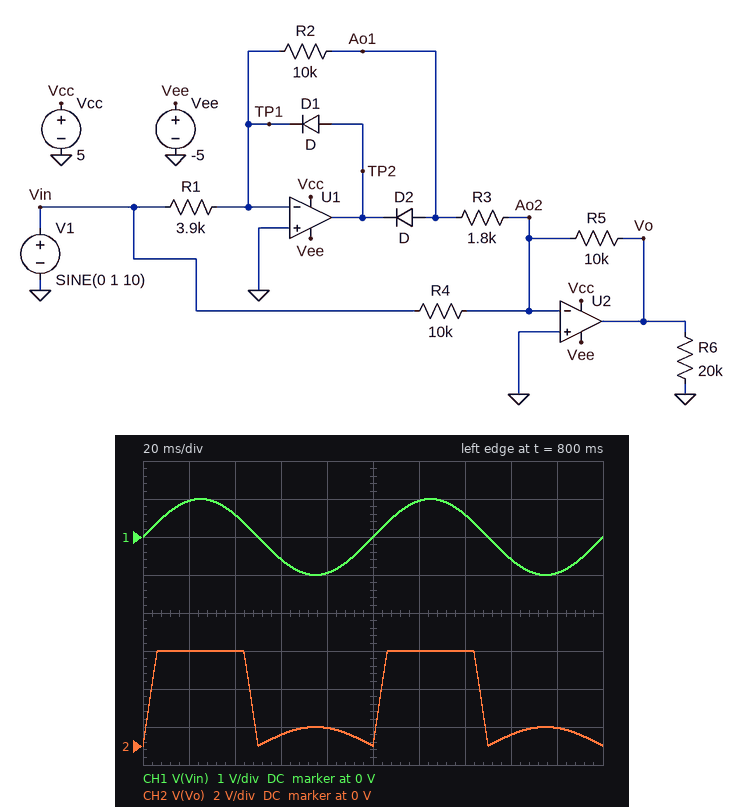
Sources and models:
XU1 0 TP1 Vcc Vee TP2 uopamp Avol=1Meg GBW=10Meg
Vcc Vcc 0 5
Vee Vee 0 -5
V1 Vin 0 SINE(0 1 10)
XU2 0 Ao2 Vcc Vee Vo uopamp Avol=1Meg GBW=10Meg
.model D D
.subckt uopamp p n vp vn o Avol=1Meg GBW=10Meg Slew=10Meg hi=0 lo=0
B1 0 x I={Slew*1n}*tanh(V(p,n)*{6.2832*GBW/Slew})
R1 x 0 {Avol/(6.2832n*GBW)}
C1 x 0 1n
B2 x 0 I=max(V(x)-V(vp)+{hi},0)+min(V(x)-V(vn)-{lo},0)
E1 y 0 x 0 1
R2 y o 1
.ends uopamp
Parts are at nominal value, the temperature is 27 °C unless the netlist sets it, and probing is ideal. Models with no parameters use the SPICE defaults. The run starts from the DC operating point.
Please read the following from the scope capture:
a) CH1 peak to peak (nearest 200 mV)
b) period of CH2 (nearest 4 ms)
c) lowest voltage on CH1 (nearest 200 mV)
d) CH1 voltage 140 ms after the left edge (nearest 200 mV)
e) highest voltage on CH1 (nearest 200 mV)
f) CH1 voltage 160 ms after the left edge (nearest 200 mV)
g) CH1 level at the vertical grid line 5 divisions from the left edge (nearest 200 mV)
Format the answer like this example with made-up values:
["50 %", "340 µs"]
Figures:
["2.0 V", "100 ms", "-1.0 V", "600 mV", "1.0 V", "-600 mV", "0 V"]
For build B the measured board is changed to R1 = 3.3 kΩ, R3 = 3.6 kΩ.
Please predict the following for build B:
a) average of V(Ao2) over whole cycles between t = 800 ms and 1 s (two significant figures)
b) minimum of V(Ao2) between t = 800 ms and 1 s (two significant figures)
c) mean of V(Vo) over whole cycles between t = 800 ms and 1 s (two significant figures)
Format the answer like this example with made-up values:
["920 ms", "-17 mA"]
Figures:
["-88 mV", "-500 mV", "2.3 V"]
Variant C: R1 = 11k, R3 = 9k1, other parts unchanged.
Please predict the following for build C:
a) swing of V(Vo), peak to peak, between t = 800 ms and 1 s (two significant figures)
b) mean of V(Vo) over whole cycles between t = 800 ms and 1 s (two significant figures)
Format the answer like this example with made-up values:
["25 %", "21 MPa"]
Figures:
["1.0 V", "320 mV"]
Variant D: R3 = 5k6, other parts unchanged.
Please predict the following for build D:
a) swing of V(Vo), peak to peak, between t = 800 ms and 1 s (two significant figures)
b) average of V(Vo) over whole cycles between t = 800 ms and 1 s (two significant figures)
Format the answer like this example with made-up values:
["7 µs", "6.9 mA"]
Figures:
["3.6 V", "1.5 V"]
